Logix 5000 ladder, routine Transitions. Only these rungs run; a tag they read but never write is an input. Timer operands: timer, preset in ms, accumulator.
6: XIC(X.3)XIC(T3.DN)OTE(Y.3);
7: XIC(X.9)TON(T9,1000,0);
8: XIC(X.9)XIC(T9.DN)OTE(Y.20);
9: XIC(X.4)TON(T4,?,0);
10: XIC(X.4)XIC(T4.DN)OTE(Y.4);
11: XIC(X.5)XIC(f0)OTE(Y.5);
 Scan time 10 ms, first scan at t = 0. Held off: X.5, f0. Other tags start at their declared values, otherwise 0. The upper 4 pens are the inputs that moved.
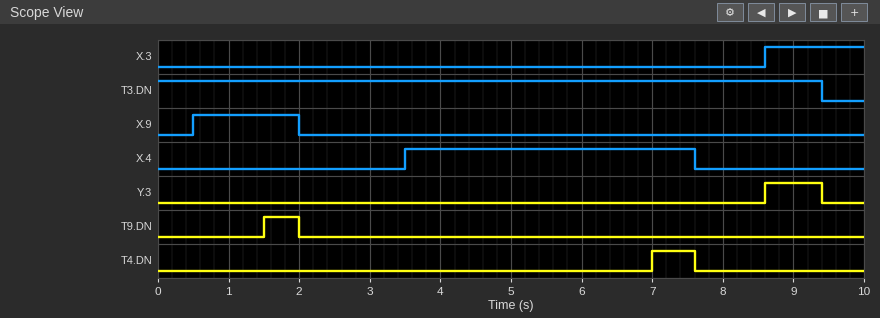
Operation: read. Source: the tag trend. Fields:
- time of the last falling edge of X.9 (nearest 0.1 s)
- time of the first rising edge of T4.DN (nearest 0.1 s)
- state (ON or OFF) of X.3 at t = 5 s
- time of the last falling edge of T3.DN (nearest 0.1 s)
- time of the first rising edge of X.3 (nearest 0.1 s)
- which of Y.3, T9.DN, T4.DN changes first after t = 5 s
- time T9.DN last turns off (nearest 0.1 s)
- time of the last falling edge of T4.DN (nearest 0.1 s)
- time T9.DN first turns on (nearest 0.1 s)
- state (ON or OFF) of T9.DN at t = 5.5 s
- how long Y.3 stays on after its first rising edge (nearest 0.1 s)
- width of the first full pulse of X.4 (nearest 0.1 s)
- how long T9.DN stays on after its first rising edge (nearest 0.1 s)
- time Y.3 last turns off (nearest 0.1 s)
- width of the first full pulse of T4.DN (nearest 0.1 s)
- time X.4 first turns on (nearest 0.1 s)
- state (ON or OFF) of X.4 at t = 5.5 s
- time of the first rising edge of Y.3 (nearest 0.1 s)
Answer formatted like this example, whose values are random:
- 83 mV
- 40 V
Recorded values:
- 2.0 s
- 7.0 s
- OFF
- 9.4 s
- 8.6 s
- T4.DN
- 2.0 s
- 7.6 s
- 1.5 s
- OFF
- 0.8 s
- 4.1 s
- 0.5 s
- 9.4 s
- 0.6 s
- 3.5 s
- ON
- 8.6 s
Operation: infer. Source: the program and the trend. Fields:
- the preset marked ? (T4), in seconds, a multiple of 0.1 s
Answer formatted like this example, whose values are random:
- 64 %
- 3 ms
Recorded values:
- 3.5 s
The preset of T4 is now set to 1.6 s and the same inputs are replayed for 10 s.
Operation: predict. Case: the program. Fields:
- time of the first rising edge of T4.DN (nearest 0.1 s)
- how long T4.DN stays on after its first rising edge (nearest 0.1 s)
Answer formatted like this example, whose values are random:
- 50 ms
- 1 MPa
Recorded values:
- 5.1 s
- 2.5 s
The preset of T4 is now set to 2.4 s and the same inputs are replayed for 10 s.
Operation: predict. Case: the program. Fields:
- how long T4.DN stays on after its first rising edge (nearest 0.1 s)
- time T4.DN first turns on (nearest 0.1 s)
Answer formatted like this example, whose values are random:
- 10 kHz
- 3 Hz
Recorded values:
- 1.7 s
- 5.9 s
